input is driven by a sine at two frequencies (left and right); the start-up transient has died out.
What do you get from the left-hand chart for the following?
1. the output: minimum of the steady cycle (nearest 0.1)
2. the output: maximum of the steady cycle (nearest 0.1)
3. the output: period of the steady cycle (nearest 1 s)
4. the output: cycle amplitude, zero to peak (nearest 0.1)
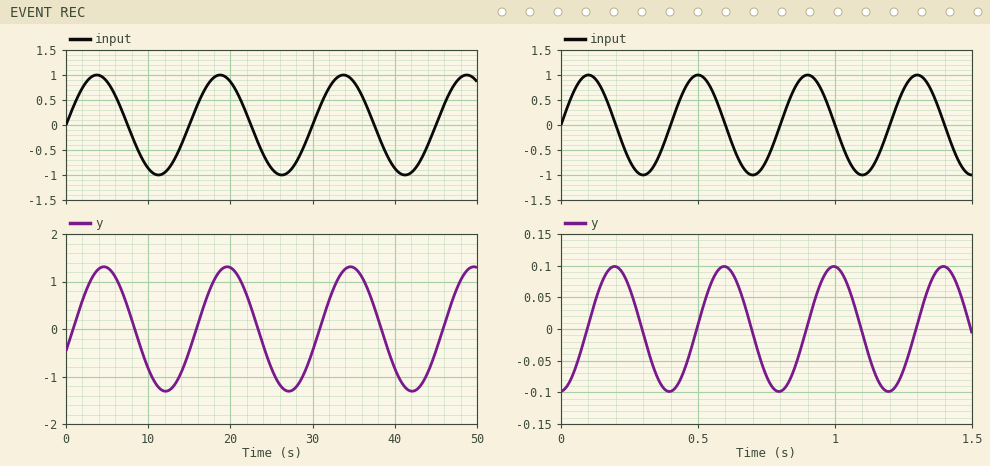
-1.3
1.3
15 s
1.3
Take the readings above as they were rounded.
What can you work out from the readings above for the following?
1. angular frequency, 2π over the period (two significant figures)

0.42 rad/s
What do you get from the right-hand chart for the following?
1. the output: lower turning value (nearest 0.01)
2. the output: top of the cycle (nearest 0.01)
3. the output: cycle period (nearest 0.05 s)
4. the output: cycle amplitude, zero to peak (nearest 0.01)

-0.10
0.10
0.40 s
0.10
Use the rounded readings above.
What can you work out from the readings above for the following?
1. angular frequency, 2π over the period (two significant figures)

16 rad/s
